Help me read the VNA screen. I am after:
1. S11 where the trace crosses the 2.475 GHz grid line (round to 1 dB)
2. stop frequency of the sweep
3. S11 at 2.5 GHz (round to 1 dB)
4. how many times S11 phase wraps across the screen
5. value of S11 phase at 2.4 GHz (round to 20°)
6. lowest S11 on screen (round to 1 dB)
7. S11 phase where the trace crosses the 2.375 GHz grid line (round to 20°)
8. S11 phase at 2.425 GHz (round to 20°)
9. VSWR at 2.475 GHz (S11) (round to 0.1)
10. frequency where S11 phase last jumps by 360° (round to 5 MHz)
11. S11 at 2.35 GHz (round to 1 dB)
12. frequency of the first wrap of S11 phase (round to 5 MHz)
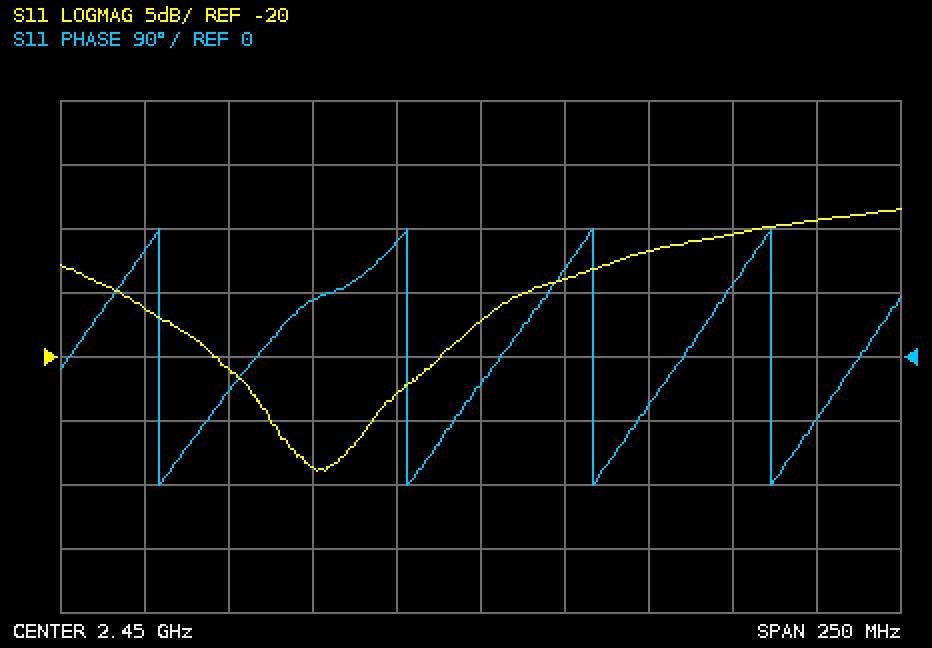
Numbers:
-14 dB
2.575 GHz
-12 dB
4
80°
-29 dB
-40°
160°
1.5
2.535 GHz
-16 dB
2.355 GHz
